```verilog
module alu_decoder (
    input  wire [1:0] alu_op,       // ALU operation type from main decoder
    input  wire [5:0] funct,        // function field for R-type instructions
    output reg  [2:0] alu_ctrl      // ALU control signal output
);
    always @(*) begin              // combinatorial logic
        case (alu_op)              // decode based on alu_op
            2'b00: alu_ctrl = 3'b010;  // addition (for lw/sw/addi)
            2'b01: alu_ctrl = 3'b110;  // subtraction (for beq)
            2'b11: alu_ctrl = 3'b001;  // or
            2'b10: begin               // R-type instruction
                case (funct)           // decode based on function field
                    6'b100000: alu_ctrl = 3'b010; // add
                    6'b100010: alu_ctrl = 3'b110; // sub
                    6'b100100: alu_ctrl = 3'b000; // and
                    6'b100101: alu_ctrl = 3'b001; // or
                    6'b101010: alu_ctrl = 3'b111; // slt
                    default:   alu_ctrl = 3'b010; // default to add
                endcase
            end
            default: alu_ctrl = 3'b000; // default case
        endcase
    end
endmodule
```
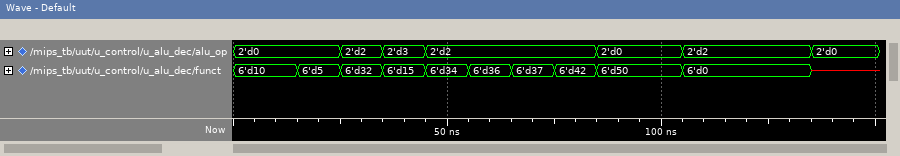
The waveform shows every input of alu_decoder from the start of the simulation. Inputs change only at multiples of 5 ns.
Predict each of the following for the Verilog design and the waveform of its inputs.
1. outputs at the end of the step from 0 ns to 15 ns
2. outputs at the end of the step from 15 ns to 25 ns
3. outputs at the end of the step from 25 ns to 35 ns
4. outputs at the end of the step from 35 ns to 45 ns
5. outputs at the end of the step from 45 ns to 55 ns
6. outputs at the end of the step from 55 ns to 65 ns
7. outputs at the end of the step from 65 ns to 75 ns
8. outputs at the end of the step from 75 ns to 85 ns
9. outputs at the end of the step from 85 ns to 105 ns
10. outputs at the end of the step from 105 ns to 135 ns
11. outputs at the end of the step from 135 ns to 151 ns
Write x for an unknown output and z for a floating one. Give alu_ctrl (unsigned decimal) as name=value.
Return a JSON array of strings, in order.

["alu_ctrl=2", "alu_ctrl=2", "alu_ctrl=2", "alu_ctrl=1", "alu_ctrl=6", "alu_ctrl=0", "alu_ctrl=1", "alu_ctrl=7", "alu_ctrl=2", "alu_ctrl=2", "alu_ctrl=2"]
